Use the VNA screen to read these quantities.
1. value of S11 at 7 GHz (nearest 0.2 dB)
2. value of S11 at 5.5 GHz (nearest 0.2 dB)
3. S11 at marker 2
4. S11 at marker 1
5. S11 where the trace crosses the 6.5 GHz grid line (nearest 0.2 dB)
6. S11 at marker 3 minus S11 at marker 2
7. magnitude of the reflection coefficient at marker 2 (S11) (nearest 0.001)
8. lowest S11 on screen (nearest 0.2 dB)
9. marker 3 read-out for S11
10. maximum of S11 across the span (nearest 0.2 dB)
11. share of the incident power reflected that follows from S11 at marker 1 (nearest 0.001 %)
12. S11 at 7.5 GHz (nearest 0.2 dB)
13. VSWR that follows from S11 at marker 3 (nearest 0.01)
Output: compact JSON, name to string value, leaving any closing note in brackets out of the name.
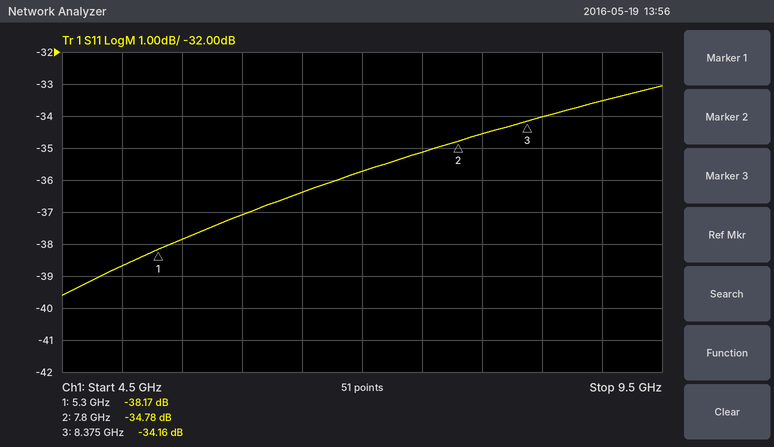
{"value of S11 at 7 GHz": "-35.8 dB", "value of S11 at 5.5 GHz": "-37.8 dB", "S11 at marker 2": "-34.78 dB", "S11 at marker 1": "-38.17 dB", "S11 where the trace crosses the 6.5 GHz grid line": "-36.4 dB", "S11 at marker 3 minus S11 at marker 2": "0.62 dB", "magnitude of the reflection coefficient at marker 2 (S11)": "0.018", "lowest S11 on screen": "-39.6 dB", "marker 3 read-out for S11": "-34.16 dB", "maximum of S11 across the span": "-33.0 dB", "share of the incident power reflected that follows from S11 at marker 1": "0.015 %", "S11 at 7.5 GHz": "-35.2 dB", "VSWR that follows from S11 at marker 3": "1.04"}
